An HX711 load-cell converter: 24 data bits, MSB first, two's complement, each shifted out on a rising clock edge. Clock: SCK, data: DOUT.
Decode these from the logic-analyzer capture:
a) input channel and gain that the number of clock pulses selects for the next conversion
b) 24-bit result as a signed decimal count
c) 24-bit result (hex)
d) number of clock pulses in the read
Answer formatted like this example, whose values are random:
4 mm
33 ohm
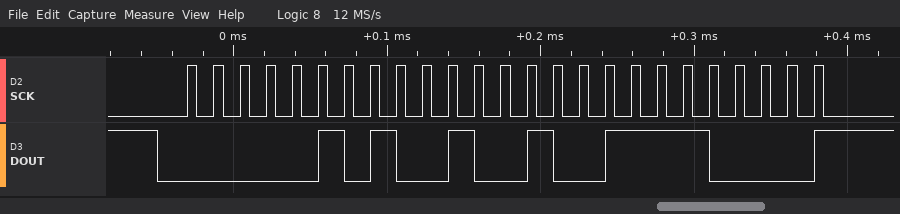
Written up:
channel A, gain 128
337136
0x0524F0
25
